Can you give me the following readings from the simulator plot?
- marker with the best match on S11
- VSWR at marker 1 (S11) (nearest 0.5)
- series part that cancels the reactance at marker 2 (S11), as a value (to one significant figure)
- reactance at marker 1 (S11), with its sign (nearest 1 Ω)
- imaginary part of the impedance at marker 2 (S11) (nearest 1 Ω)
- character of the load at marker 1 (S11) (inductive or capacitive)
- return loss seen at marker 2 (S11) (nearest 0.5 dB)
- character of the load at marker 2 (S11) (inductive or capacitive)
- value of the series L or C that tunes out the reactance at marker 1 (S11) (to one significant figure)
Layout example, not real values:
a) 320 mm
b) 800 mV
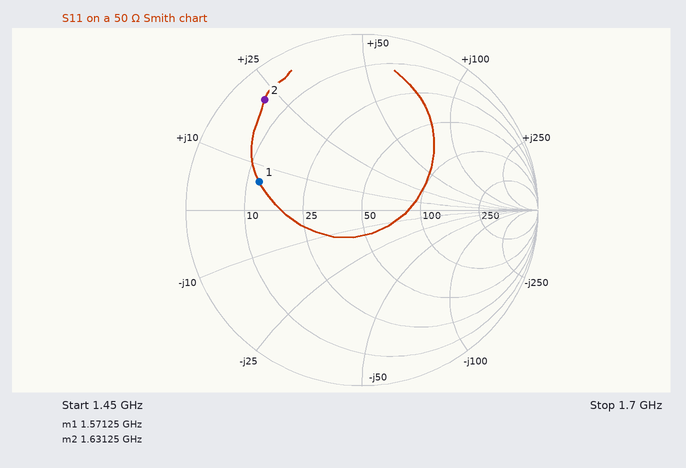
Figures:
a) marker 1
b) 4.0
c) 4 pF
d) +6 Ω
e) +22 Ω
f) inductive
g) 1.5 dB
h) inductive
i) 20 pF
